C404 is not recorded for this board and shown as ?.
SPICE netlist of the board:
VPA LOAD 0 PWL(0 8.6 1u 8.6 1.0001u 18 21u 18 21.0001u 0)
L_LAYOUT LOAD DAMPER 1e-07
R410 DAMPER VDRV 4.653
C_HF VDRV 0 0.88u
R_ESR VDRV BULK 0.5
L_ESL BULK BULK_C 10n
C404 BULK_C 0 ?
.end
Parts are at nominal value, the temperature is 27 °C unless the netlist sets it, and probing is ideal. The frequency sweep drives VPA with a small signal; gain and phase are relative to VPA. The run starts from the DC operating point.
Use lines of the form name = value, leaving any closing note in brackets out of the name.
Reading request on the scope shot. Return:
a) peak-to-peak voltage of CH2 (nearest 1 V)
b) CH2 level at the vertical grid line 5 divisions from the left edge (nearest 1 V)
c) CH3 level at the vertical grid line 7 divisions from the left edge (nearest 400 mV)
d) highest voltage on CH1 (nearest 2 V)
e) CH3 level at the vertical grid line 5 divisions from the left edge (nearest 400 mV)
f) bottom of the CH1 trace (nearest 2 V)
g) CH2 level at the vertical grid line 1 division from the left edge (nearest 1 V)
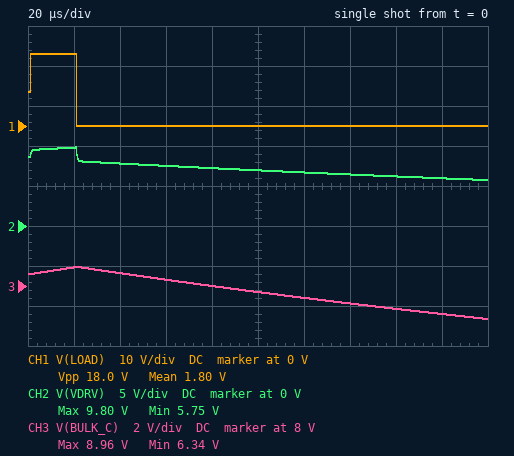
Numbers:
peak-to-peak voltage of CH2 = 4 V
CH2 level at the vertical grid line 5 divisions from the left edge = 7 V
CH3 level at the vertical grid line 7 divisions from the left edge = 7.2 V
highest voltage on CH1 = 18 V
CH3 level at the vertical grid line 5 divisions from the left edge = 7.6 V
bottom of the CH1 trace = 0 V
CH2 level at the vertical grid line 1 division from the left edge = 10 V
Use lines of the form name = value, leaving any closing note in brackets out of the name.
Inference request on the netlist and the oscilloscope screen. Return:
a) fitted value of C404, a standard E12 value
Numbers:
fitted value of C404, a standard E12 value = 100 µF
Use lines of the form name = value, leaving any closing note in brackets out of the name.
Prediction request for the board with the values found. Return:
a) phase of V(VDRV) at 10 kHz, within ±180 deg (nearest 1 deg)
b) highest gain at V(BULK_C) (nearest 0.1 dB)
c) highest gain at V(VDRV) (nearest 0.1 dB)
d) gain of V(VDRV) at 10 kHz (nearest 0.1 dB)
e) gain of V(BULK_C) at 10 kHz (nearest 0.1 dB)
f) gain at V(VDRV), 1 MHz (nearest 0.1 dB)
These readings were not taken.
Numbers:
phase of V(VDRV) at 10 kHz, within ±180 deg = -17 deg
highest gain at V(BULK_C) = 0 dB
highest gain at V(VDRV) = 0 dB
gain of V(VDRV) at 10 kHz = -19.9 dB
gain of V(BULK_C) at 10 kHz = -30.3 dB
gain at V(VDRV), 1 MHz = -28.5 dB
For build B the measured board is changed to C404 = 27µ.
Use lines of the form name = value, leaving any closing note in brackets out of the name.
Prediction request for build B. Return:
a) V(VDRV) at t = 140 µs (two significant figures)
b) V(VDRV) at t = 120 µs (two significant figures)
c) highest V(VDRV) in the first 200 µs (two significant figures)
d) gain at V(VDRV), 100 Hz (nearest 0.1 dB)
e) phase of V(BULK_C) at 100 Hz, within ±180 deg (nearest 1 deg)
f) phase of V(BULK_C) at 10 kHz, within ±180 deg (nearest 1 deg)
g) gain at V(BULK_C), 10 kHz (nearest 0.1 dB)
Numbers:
V(VDRV) at t = 140 µs = 3.9 V
V(VDRV) at t = 120 µs = 4.5 V
highest V(VDRV) in the first 200 µs = 11 V
gain at V(VDRV), 100 Hz = 0 dB
phase of V(BULK_C) at 100 Hz, within ±180 deg = -5 deg
phase of V(BULK_C) at 10 kHz, within ±180 deg = -85 deg
gain at V(BULK_C), 10 kHz = -19.1 dB
